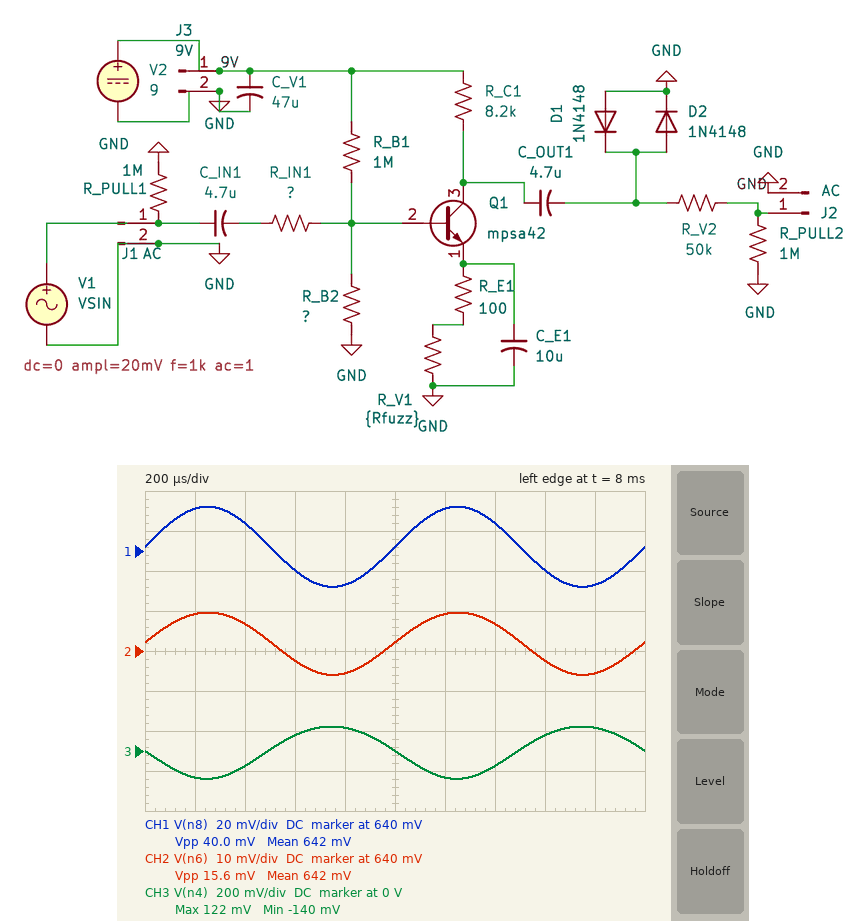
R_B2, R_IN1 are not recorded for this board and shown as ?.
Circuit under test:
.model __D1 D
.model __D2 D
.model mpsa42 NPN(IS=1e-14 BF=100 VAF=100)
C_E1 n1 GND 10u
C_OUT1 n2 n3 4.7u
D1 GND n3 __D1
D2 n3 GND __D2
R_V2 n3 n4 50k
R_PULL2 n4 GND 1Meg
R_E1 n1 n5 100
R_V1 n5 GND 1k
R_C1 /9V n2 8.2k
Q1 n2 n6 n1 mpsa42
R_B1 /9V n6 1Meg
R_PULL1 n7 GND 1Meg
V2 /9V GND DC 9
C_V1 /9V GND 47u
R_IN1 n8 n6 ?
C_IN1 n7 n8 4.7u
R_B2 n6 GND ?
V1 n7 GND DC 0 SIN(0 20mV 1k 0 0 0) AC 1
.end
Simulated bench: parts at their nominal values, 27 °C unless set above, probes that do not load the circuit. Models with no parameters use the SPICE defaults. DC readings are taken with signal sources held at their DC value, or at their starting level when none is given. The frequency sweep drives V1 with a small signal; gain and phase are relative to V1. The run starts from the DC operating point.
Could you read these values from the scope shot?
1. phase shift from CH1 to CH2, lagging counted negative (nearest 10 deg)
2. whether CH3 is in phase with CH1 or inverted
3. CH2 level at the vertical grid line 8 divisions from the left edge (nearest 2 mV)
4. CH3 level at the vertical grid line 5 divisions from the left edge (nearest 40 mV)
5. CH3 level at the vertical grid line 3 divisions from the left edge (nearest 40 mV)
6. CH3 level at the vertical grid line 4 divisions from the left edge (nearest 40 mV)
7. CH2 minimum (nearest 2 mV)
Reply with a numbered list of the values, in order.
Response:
1. 0 deg
2. inverted
3. 638 mV
4. 0 V
5. 80 mV
6. 120 mV
7. 634 mV
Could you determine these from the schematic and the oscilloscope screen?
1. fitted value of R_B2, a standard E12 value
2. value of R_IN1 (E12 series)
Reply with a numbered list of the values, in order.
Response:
1. 82 kΩ
2. 47 kΩ
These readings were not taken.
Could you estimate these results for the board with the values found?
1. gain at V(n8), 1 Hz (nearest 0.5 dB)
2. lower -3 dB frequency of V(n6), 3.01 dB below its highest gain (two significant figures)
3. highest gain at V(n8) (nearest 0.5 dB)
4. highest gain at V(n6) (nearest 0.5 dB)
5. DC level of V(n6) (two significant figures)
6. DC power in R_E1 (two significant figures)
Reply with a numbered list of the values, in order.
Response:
1. -0.5 dB
2. 340 mHz
3. 0 dB
4. -5.5 dB
5. 640 mV
6. 330 nW
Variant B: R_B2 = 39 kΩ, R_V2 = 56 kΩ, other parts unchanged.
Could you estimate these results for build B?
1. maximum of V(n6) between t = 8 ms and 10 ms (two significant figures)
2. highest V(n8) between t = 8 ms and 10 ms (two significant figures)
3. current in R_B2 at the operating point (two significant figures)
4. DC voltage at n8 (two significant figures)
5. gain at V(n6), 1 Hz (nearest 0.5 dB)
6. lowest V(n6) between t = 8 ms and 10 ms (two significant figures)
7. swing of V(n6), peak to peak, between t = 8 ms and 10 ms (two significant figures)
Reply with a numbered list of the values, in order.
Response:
1. 350 mV
2. 360 mV
3. 8.7 µA
4. 340 mV
5. -7.5 dB
6. 330 mV
7. 18 mV
